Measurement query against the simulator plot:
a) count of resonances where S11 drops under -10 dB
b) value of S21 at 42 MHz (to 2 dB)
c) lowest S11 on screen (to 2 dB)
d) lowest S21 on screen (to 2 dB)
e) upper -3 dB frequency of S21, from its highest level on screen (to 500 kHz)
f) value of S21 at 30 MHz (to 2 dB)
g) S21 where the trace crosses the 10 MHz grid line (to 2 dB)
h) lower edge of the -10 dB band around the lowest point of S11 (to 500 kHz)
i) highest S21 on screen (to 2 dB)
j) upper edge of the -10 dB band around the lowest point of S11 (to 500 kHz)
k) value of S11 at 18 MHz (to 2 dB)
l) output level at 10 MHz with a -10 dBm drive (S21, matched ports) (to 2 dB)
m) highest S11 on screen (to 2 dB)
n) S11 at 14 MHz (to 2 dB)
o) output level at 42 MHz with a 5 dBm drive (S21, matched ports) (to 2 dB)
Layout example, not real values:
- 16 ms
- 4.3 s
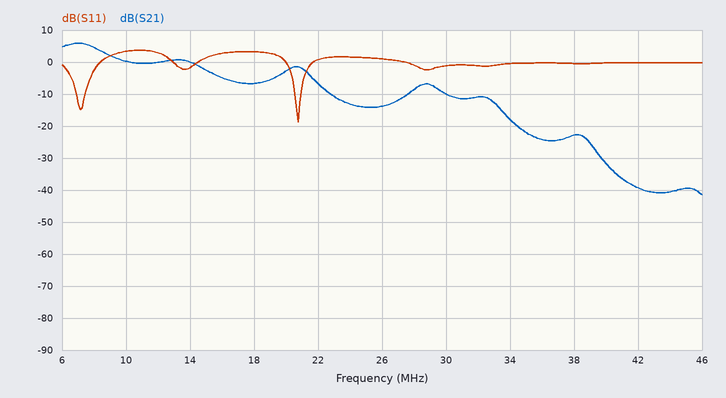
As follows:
- 2
- -40 dB
- -18 dB
- -42 dB
- 8.5 MHz
- -10 dB
- 0 dB
- 20.5 MHz
- 6 dB
- 21.0 MHz
- 4 dB
- -10 dBm
- 4 dB
- -2 dB
- -34 dBm
